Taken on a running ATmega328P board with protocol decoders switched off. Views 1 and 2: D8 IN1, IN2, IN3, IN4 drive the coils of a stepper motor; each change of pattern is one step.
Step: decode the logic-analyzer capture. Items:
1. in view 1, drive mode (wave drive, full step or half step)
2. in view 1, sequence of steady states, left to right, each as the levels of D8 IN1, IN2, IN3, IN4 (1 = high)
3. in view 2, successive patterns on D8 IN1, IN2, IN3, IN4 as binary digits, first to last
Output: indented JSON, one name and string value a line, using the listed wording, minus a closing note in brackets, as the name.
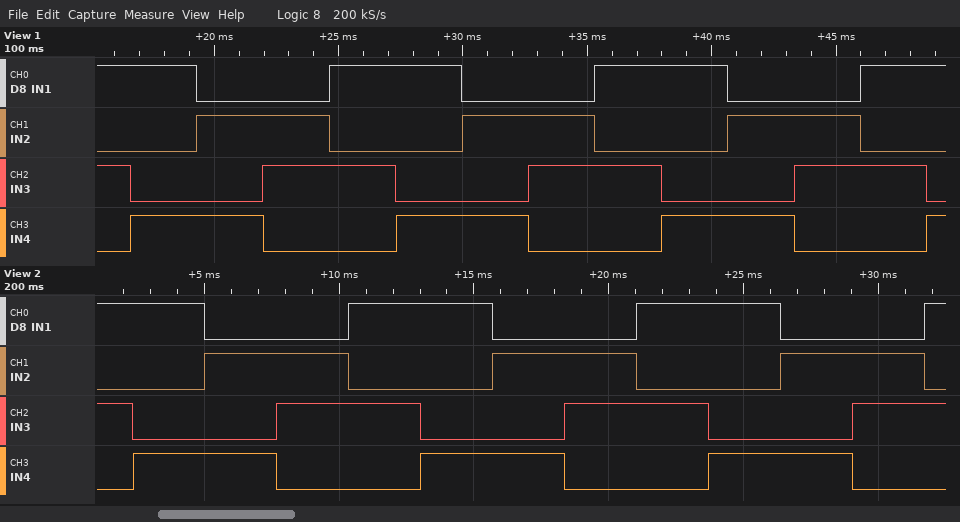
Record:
{
  "in view 1, drive mode": "full step",
  "in view 1, sequence of steady states, left to right, each as the levels of D8 IN1, IN2, IN3, IN4": "1010 1001 0101 0110 1010 1001 0101 0110 1010 1001 0101 0110 1010 1001",
  "in view 2, successive patterns on D8 IN1, IN2, IN3, IN4 as binary digits, first to last": "1010 1001 0101 0110 1010 1001 0101 0110 1010 1001 0101 0110 1010"
}
